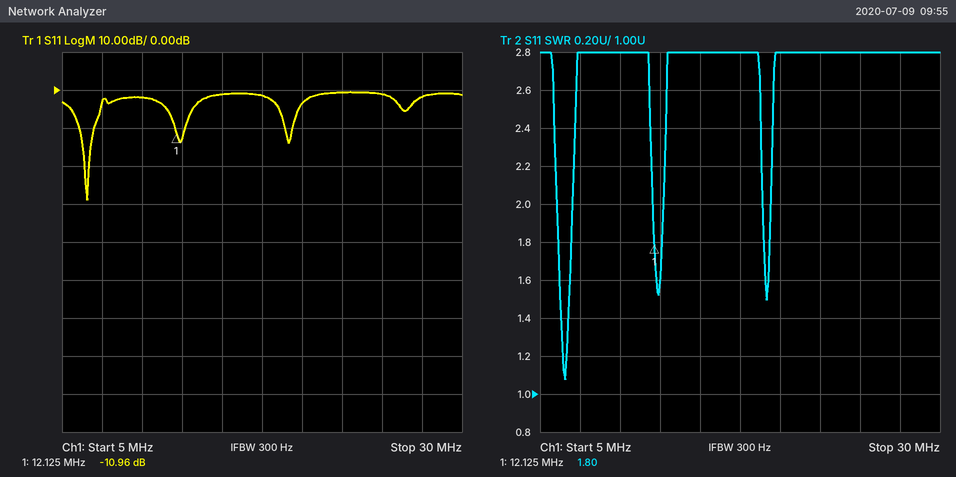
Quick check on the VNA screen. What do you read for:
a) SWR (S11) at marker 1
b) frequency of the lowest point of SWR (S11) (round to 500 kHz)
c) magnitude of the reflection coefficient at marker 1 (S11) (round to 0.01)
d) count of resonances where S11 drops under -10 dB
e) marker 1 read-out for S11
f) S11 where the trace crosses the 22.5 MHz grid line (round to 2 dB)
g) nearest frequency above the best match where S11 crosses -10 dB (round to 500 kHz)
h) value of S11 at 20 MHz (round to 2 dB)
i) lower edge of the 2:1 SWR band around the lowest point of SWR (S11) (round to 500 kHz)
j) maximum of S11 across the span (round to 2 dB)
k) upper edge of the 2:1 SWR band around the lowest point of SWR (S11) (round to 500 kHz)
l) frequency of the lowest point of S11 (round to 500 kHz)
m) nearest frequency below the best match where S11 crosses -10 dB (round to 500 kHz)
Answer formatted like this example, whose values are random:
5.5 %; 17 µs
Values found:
1.80; 6.5 MHz; 0.28; 3; -10.96 dB; 0 dB; 7.0 MHz; -4 dB; 6.0 MHz; 0 dB; 7.0 MHz; 6.5 MHz; 6.0 MHz
